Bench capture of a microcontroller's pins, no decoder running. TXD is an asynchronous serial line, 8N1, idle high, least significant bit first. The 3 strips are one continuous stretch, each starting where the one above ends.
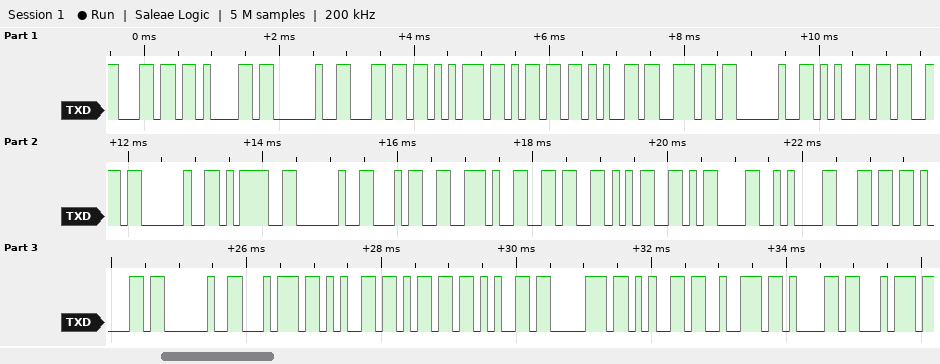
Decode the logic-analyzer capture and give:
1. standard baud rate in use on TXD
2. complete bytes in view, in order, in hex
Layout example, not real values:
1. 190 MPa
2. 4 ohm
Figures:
1. 9600 baud
2. 0x6C 0x61 0x20 0x6C 0x75 0x6D 0x65 0x6E 0x20 0x65 0x73 0x20 0x3D 0x20 0x34 0x2E 0x36 0x35 0x0D 0x0A 0x6C 0x61 0x20 0x74 0x65 0x6D 0x65 0x70 0x65 0x72 0x61 0x74
